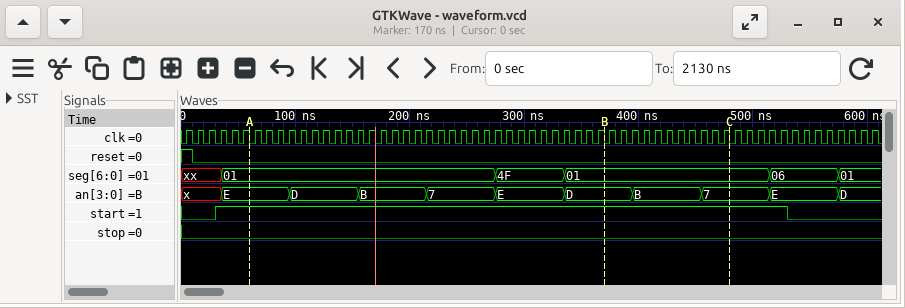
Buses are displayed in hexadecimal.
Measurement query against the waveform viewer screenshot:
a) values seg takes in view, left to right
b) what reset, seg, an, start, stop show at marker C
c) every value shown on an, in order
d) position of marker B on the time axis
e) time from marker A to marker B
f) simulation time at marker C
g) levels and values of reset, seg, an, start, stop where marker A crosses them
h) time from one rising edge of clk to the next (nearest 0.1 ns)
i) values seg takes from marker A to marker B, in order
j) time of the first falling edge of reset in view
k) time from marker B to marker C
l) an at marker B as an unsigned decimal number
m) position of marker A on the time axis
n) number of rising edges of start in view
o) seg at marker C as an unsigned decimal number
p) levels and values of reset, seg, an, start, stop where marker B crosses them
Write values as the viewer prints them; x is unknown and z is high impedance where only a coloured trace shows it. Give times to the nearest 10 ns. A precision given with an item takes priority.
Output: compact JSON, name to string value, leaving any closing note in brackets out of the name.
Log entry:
{"values seg takes in view, left to right": "xx, 01, 4F, 01, 06, 01", "what reset, seg, an, start, stop show at marker C": "reset=0, seg=01, an=7, start=1, stop=0", "every value shown on an, in order": "x, E, D, B, 7, E, D, B, 7, E, D", "position of marker B on the time axis": "370 ns", "time from marker A to marker B": "310 ns", "simulation time at marker C": "480 ns", "levels and values of reset, seg, an, start, stop where marker A crosses them": "reset=0, seg=01, an=E, start=1, stop=0", "time from one rising edge of clk to the next": "10 ns", "values seg takes from marker A to marker B, in order": "01, 4F, 01", "time of the first falling edge of reset in view": "10 ns", "time from marker B to marker C": "110 ns", "an at marker B as an unsigned decimal number": "13", "position of marker A on the time axis": "60 ns", "number of rising edges of start in view": "1", "seg at marker C as an unsigned decimal number": "1", "levels and values of reset, seg, an, start, stop where marker B crosses them": "reset=0, seg=01, an=D, start=1, stop=0"}
